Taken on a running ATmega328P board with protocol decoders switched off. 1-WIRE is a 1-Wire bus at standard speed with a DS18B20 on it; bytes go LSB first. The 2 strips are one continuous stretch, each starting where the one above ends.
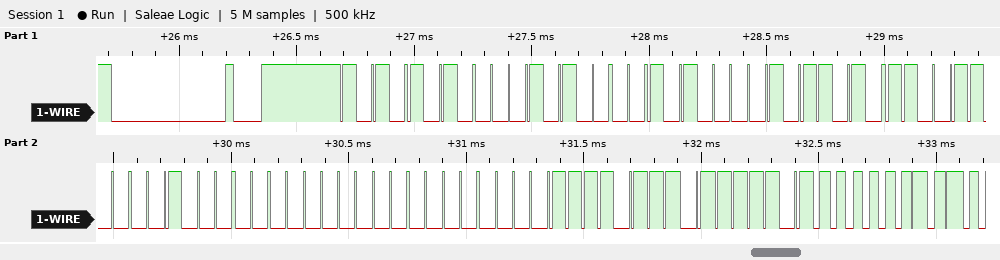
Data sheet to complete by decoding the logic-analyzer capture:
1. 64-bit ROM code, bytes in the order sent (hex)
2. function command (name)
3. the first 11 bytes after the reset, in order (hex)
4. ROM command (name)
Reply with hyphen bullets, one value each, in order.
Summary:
- 28 14 5A 33 04 00 00 EF
- Read Scratchpad
- 55 28 14 5A 33 04 00 00 EF BE 40
- Match ROM
